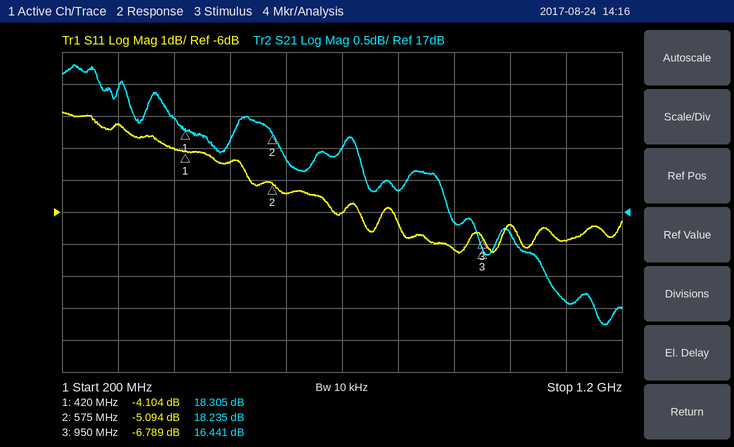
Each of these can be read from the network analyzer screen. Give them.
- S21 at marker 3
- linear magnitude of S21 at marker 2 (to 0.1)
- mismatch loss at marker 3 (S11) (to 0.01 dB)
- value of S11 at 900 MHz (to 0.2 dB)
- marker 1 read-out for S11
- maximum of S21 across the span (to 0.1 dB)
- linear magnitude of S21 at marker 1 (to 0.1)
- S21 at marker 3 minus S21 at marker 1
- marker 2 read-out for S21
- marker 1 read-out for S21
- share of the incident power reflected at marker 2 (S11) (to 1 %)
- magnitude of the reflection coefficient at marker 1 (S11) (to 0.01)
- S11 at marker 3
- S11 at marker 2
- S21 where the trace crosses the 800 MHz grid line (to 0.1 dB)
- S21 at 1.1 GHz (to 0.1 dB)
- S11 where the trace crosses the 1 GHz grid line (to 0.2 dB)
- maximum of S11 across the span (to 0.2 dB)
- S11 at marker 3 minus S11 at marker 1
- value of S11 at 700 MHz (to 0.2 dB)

16.441 dB
8.2
1.02 dB
-7.2 dB
-4.104 dB
19.3 dB
8.2
-1.864 dB
18.235 dB
18.305 dB
31 %
0.62
-6.789 dB
-5.094 dB
17.3 dB
15.6 dB
-6.4 dB
-2.8 dB
-2.685 dB
-6.0 dB
